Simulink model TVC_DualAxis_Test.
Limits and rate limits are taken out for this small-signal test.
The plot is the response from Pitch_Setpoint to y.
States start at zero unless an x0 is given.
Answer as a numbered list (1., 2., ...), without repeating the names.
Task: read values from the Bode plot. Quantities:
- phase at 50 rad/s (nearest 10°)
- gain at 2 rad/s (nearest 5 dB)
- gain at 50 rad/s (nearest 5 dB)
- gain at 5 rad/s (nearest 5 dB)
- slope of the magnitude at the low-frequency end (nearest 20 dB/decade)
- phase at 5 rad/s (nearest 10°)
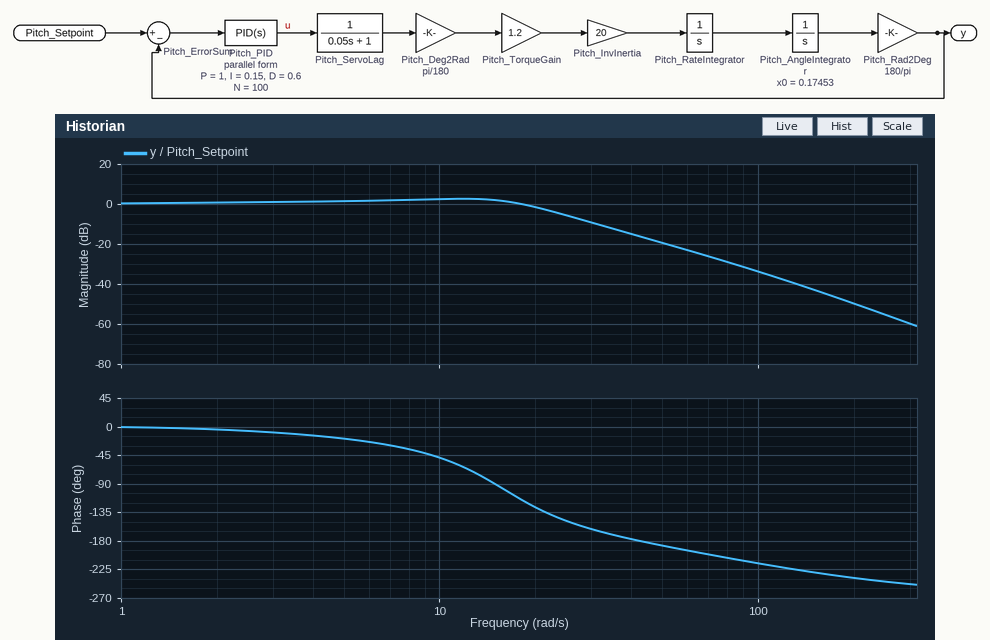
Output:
1. -190°
2. 0 dB
3. -20 dB
4. 0 dB
5. 0 dB/decade
6. -20°
